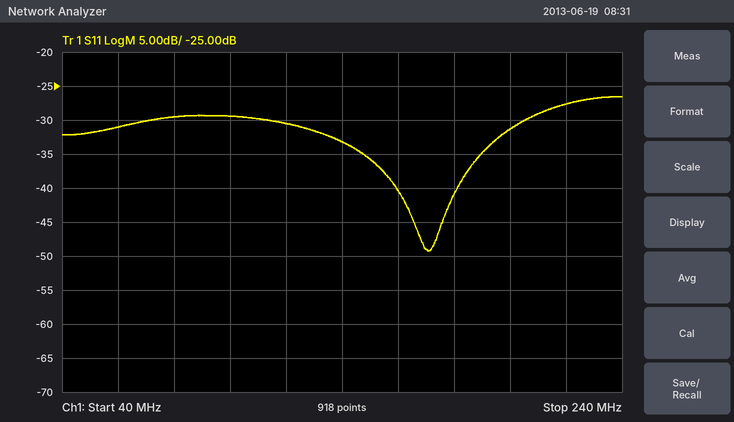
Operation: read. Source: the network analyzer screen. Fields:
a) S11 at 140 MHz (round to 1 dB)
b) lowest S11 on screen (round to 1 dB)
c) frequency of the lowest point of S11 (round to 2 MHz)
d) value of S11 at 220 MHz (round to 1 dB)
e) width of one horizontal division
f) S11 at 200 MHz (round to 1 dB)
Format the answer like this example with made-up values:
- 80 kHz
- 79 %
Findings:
- -33 dB
- -49 dB
- 170 MHz
- -28 dB
- 20 MHz
- -31 dB
